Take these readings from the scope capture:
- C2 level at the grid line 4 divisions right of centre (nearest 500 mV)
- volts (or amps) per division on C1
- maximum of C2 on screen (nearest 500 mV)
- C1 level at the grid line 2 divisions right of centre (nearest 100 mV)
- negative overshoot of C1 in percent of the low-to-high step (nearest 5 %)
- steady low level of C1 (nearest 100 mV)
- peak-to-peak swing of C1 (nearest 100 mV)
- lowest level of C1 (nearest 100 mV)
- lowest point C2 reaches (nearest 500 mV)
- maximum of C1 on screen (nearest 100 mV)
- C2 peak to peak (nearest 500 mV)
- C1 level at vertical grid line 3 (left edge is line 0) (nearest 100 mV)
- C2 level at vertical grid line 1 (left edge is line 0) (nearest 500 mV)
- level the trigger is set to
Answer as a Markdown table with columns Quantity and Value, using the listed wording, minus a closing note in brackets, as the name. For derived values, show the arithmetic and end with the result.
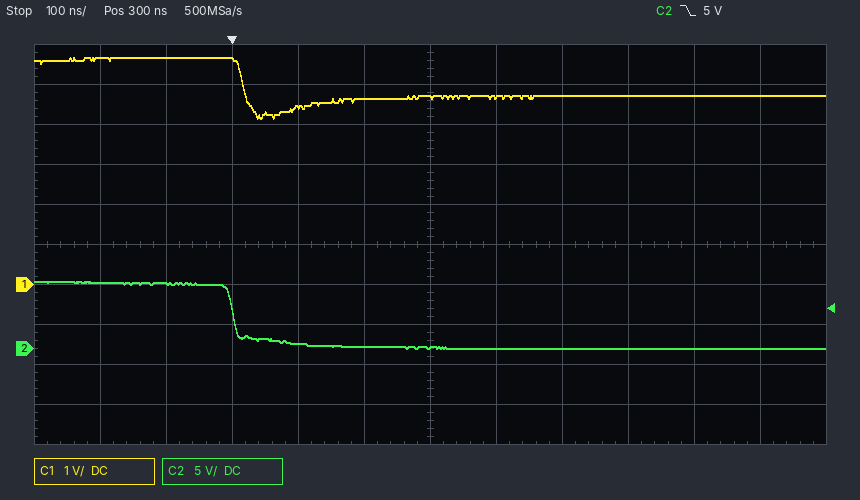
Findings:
| Quantity | Value |
|---|---|
| C2 level at the grid line 4 divisions right of centre | 0.0 V |
| volts (or amps) per division on C1 | 1 V |
| maximum of C2 on screen | 8.5 V |
| C1 level at the grid line 2 divisions right of centre | 4.7 V |
| negative overshoot of C1 in percent of the low-to-high step | 60 % |
| steady low level of C1 | 4.7 V |
| peak-to-peak swing of C1 | 5.7 V − (4.2 V) = 1.5 V |
| lowest level of C1 | 4.2 V |
| lowest point C2 reaches | 0.0 V |
| maximum of C1 on screen | 5.7 V |
| C2 peak to peak | 8.5 V − (0.0 V) = 8.5 V |
| C1 level at vertical grid line 3 (left edge is line 0) | 5.6 V |
| C2 level at vertical grid line 1 (left edge is line 0) | 8.0 V |
| level the trigger is set to | 5 V |
